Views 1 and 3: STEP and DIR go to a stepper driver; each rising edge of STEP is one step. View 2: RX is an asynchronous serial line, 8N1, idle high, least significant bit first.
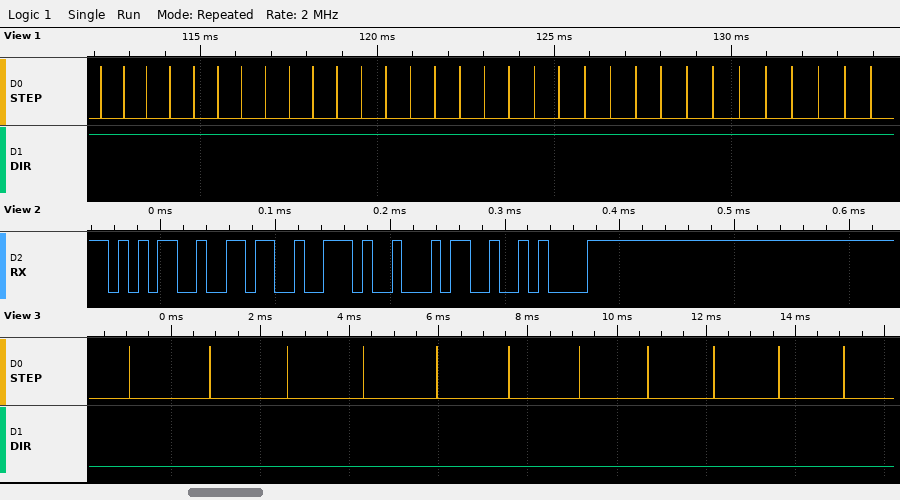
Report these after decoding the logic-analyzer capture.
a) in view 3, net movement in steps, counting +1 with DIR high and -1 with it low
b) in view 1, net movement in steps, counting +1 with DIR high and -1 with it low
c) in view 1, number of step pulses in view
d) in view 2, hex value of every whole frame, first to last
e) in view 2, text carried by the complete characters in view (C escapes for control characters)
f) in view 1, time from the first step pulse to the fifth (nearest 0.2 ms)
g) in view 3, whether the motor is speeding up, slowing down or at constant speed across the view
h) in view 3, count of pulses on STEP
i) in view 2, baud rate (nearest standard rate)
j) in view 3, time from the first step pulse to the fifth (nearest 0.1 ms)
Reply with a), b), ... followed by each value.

a) -11
b) +32
c) 32
d) 0x35 0x36 0x2E 0x34 0x0A
e) "56.4\n"
f) 2.6 ms
g) speeding up
h) 11
i) 115200 baud
j) 6.9 ms
